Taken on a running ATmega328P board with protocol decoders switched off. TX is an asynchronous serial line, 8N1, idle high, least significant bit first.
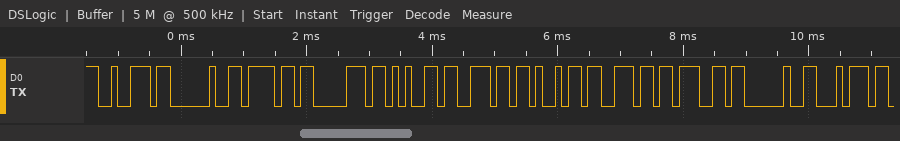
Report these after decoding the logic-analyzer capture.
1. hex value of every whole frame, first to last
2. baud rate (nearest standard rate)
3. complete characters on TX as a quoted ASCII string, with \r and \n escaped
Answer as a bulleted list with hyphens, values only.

- 0x72 0x20 0x6F 0x70 0x65 0x6E 0x69 0x6E 0x67 0x20 0x74
- 9600 baud
- "r opening t"
